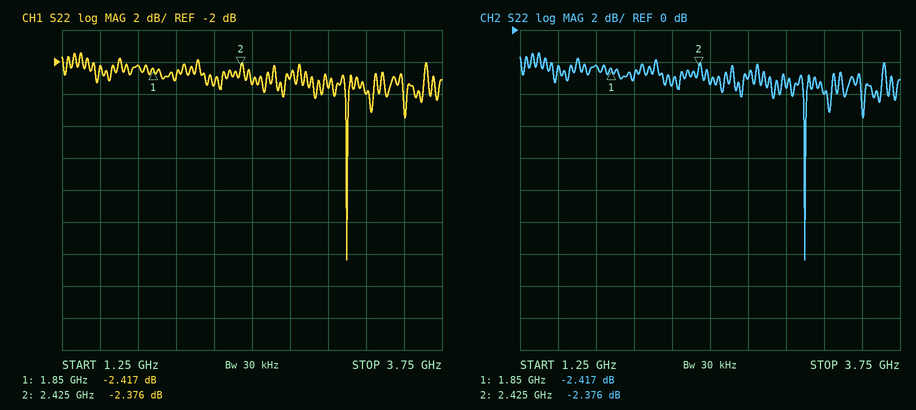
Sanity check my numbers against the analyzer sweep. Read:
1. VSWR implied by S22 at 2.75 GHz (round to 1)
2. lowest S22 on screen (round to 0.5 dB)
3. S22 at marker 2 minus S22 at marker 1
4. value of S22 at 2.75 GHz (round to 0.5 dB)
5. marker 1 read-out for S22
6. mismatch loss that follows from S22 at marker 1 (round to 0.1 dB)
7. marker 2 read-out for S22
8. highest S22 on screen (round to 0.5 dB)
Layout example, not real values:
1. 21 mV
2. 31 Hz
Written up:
1. 6
2. -14.5 dB
3. 0.041 dB
4. -3.0 dB
5. -2.417 dB
6. 3.7 dB
7. -2.376 dB
8. -1.5 dB
